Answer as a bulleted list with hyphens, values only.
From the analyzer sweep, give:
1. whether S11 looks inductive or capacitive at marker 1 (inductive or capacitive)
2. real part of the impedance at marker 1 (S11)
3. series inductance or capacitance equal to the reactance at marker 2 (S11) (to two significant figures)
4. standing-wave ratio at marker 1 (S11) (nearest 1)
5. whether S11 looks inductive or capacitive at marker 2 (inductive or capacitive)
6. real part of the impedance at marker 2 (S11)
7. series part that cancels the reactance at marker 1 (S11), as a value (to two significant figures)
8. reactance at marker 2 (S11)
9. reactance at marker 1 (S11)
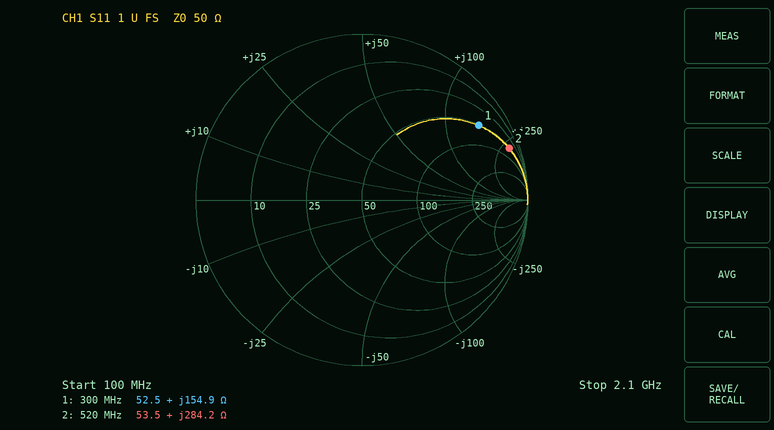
- inductive
- 52.5 Ω
- 87 nH
- 11
- inductive
- 53.5 Ω
- 3.4 pF
- +284.2 Ω
- +154.9 Ω
